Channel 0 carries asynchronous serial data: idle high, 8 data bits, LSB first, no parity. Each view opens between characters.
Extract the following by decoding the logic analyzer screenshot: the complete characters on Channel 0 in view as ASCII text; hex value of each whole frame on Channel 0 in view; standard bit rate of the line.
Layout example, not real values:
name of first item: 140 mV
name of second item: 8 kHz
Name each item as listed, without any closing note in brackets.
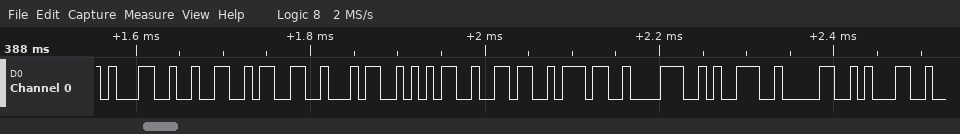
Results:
the complete characters on Channel 0 in view as ASCII text: "12345678901"
hex value of each whole frame on Channel 0 in view: 31, 32, 33, 34, 35, 36, 37, 38, 39, 30, 31
standard bit rate of the line: 115200 baud
